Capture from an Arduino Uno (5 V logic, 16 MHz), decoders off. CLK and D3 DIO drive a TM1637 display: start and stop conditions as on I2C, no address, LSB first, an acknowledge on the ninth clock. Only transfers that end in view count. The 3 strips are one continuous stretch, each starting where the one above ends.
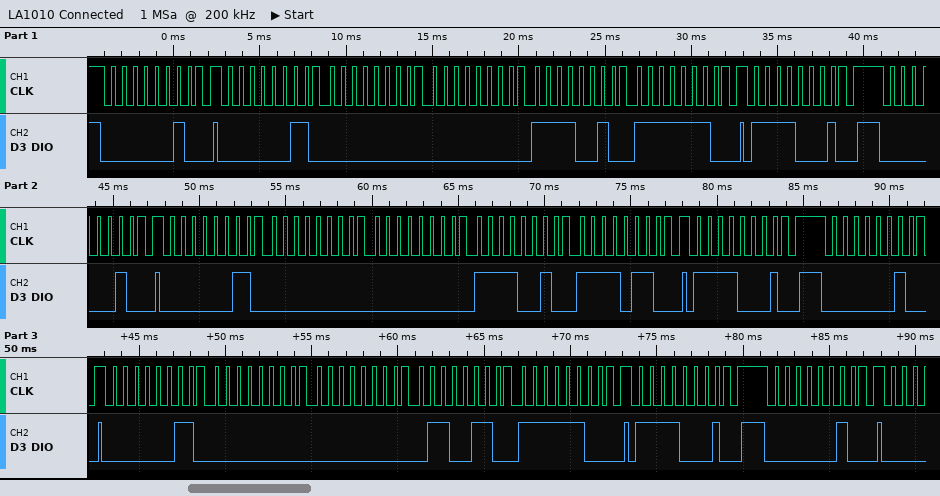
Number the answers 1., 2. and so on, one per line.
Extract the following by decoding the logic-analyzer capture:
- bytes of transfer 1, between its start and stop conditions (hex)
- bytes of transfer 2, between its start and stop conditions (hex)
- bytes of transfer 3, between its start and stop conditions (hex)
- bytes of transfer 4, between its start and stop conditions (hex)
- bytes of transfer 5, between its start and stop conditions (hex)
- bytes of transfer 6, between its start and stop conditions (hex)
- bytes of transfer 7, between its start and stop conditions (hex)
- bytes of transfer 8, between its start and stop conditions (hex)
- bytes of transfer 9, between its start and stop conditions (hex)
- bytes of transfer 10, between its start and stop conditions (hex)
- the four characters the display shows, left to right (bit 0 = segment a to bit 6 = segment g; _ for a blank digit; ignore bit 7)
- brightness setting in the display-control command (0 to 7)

1. 40
2. C0 00 00 4F 7F
3. 8F
4. 40
5. C0 00 00 4F 6F
6. 8F
7. 40
8. C0 00 00 66 3F
9. 8F
10. 40
11. __40
12. 7
